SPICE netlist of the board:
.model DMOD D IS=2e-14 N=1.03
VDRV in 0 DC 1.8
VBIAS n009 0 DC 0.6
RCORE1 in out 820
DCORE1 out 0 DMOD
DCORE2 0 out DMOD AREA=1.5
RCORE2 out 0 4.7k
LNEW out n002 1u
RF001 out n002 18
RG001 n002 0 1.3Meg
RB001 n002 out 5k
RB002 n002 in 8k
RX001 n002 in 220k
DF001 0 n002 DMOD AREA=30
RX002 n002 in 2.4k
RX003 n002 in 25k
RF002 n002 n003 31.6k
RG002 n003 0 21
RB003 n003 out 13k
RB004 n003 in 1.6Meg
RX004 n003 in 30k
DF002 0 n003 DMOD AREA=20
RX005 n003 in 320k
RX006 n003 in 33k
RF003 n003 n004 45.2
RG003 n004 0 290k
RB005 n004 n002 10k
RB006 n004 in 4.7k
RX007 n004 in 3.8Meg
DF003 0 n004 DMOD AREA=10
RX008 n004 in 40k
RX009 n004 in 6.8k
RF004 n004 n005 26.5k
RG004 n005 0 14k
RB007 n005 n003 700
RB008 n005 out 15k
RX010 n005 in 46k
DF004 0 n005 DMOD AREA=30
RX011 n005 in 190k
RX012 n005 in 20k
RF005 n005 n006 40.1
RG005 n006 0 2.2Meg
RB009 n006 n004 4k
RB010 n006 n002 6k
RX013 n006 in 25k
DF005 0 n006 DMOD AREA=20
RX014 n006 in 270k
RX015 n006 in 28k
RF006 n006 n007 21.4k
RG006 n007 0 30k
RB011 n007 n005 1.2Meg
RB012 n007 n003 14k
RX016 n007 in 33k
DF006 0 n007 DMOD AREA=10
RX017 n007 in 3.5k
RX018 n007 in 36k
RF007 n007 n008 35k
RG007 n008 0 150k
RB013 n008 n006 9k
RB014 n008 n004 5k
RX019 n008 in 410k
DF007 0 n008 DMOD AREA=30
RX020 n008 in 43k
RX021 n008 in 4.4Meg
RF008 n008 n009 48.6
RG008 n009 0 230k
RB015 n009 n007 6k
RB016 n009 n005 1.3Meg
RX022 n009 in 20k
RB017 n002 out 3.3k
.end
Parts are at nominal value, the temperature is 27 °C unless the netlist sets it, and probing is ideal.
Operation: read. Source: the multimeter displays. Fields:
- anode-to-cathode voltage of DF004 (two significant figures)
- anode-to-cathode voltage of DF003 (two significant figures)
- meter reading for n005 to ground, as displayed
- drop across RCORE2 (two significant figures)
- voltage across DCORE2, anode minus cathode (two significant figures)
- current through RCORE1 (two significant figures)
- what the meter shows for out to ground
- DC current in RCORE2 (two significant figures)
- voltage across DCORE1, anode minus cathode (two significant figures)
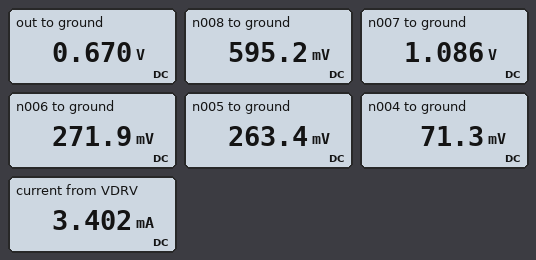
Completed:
-260 mV
-71 mV
263.4 mV
670 mV
-670 mV
1.4 mA
0.670 V
140 µA
670 mV
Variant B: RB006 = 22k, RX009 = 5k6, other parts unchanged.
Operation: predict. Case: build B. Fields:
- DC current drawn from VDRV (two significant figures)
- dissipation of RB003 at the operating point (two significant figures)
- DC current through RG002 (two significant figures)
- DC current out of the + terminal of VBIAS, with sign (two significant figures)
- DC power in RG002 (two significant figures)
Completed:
3.2 mA
32 µW
1.3 mA
-35 µA
33 µW
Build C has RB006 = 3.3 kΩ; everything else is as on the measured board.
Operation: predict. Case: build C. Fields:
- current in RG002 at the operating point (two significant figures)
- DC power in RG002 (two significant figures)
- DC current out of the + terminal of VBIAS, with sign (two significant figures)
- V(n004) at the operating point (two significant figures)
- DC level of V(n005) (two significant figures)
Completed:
1.6 mA
56 µW
-41 µA
81 mV
270 mV
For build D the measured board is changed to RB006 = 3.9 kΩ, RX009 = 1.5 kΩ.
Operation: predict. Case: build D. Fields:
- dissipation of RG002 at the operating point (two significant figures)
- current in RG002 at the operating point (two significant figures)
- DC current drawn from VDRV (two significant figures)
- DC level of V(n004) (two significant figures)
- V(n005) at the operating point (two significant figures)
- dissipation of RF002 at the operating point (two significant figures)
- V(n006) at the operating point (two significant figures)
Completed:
120 µW
2.4 mA
4.3 mA
130 mV
280 mV
12 µW
290 mV
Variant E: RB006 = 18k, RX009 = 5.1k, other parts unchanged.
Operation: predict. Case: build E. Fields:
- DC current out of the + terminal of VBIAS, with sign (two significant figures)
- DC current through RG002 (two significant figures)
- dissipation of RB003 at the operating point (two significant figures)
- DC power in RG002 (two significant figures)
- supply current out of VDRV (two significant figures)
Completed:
-36 µA
1.3 mA
32 µW
36 µW
3.2 mA
